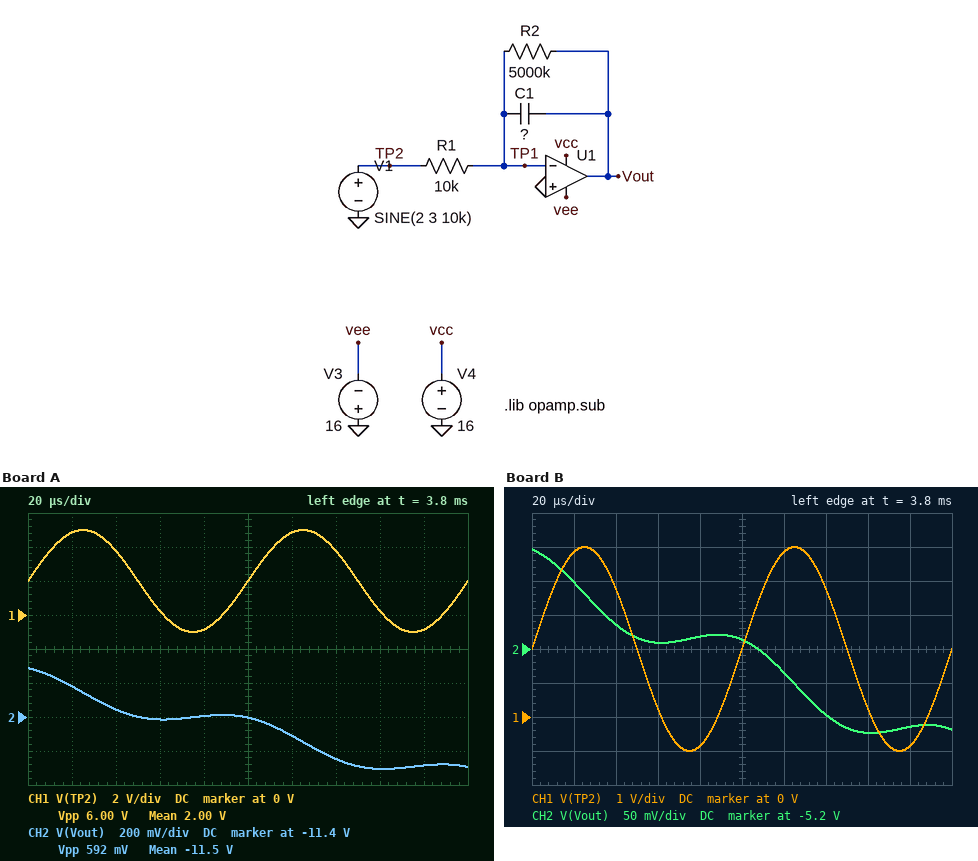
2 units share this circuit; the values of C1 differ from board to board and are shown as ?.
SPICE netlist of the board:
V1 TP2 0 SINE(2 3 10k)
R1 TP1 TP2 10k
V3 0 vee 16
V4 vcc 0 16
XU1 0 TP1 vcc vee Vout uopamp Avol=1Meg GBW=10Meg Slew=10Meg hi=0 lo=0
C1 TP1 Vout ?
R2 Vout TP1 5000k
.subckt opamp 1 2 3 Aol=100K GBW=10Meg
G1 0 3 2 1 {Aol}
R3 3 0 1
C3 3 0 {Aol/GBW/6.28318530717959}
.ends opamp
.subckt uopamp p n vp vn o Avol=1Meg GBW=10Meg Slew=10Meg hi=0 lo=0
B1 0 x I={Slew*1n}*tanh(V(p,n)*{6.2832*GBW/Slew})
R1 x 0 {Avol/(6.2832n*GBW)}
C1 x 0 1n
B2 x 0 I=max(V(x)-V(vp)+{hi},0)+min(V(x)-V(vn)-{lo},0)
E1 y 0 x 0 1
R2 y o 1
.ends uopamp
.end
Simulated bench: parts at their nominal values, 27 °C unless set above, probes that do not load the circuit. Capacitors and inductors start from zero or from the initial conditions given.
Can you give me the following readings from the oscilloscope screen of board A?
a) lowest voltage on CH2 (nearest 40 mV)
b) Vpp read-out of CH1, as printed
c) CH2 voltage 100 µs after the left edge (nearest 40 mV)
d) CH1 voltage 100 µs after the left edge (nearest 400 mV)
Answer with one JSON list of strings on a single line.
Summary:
["-11.72 V", "6.00 V", "-11.40 V", "2.0 V"]
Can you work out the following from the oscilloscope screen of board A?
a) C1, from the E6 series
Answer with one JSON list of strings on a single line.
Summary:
["68 nF"]
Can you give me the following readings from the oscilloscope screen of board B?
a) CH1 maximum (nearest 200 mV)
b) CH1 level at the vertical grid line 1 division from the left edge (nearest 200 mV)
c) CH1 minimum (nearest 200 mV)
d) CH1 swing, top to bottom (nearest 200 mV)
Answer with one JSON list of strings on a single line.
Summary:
["5.0 V", "4.8 V", "-1.0 V", "6.0 V"]
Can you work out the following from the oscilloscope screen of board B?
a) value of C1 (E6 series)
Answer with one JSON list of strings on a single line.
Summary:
["150 nF"]
